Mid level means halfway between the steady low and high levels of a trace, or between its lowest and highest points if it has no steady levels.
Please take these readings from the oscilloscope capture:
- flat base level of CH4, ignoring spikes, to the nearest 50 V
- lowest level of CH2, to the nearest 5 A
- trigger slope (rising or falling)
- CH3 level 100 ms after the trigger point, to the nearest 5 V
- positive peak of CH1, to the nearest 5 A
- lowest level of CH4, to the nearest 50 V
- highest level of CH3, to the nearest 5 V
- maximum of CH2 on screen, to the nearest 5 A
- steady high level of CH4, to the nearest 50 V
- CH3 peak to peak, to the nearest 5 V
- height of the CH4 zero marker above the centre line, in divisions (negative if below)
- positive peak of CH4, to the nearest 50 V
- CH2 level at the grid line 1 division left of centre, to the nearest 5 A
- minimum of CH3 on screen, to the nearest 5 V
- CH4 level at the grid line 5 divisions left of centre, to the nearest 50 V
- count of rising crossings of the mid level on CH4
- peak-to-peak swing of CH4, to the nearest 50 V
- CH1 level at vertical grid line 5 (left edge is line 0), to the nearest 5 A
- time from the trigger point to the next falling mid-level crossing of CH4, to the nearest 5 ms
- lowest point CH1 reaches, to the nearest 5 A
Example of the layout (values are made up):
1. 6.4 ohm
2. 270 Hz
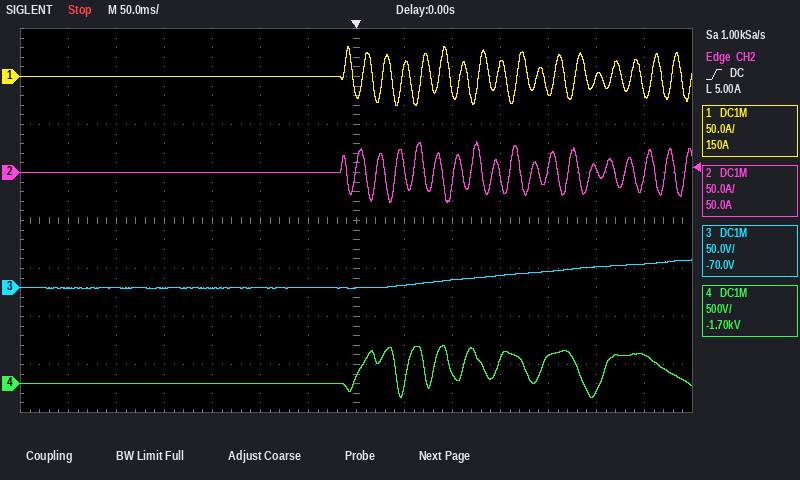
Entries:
1. 0 V
2. -30 A
3. rising
4. 10 V
5. 30 A
6. -150 V
7. 30 V
8. 30 A
9. 300 V
10. 30 V
11. -3.4 div
12. 400 V
13. 0 A
14. 0 V
15. 0 V
16. 7
17. 550 V
18. 0 A
19. 40 ms
20. -30 A
